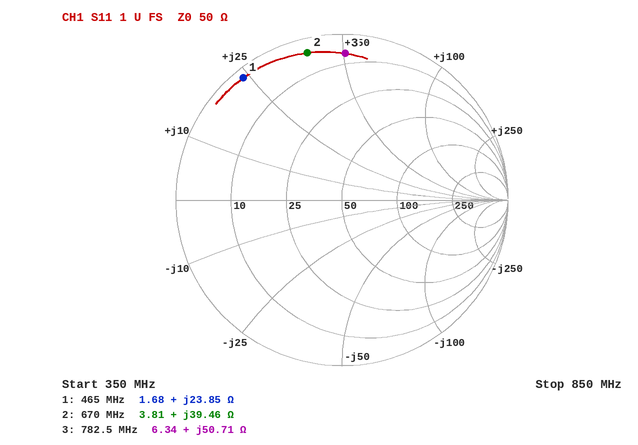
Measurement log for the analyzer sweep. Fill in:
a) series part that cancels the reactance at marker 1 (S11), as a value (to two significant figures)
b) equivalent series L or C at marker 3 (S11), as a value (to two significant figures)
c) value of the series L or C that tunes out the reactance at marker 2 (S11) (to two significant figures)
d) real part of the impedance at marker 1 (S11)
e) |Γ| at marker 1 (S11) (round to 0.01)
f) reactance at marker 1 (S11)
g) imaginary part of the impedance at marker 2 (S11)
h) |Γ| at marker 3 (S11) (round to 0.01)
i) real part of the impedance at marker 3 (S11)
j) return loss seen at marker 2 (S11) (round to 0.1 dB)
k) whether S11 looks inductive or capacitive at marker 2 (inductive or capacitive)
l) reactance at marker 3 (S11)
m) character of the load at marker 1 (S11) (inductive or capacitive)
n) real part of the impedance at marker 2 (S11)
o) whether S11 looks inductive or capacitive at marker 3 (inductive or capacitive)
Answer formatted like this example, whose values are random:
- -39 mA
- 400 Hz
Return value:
- 14 pF
- 10 nH
- 6.0 pF
- 1.68 Ω
- 0.95
- +23.85 Ω
- +39.46 Ω
- 0.88
- 6.34 Ω
- 0.8 dB
- inductive
- +50.71 Ω
- inductive
- 3.81 Ω
- inductive
